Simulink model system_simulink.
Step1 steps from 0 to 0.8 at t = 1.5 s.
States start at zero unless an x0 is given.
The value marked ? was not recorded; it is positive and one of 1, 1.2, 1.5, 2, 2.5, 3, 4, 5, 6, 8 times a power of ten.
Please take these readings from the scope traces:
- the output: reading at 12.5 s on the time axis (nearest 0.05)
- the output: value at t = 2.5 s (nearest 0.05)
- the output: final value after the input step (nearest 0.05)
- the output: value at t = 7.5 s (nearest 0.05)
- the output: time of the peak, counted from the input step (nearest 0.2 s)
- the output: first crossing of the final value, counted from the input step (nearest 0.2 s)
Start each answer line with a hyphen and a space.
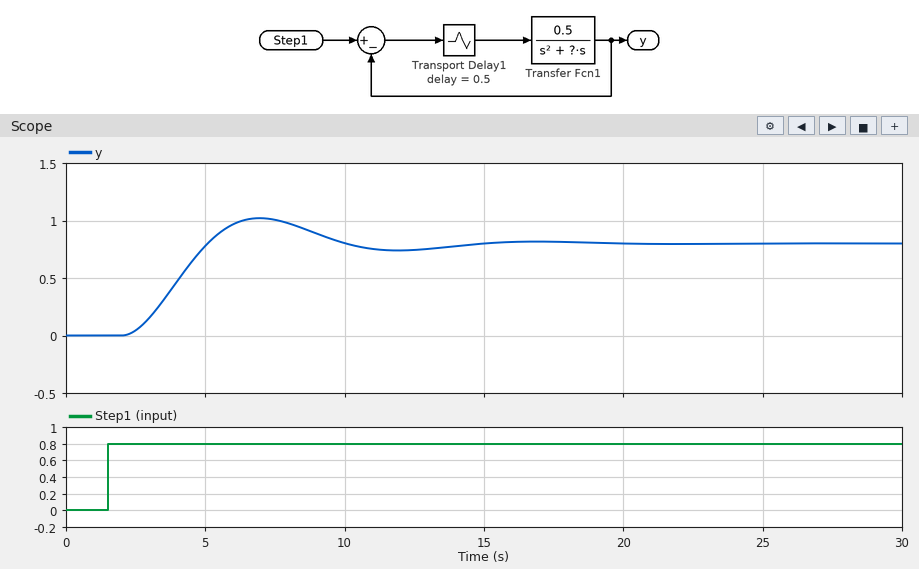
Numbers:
- 0.75
- 0.05
- 0.80
- 1.00
- 5.4 s
- 3.6 s
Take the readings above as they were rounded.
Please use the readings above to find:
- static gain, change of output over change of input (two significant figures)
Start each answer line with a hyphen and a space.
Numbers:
- 1.0
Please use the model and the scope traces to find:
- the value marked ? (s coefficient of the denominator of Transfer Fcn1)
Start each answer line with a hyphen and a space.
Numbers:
- 0.8
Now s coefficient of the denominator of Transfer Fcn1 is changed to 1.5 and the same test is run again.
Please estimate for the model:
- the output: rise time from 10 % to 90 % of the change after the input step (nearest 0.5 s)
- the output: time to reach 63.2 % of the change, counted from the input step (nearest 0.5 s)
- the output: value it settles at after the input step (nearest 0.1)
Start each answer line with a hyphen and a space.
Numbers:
- 4.0 s
- 3.5 s
- 0.8
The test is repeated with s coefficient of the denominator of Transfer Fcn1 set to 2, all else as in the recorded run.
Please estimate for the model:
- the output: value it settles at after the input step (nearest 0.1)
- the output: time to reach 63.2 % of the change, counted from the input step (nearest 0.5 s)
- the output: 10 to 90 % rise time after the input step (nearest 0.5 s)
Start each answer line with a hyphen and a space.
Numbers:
- 0.8
- 4.0 s
- 6.5 s
